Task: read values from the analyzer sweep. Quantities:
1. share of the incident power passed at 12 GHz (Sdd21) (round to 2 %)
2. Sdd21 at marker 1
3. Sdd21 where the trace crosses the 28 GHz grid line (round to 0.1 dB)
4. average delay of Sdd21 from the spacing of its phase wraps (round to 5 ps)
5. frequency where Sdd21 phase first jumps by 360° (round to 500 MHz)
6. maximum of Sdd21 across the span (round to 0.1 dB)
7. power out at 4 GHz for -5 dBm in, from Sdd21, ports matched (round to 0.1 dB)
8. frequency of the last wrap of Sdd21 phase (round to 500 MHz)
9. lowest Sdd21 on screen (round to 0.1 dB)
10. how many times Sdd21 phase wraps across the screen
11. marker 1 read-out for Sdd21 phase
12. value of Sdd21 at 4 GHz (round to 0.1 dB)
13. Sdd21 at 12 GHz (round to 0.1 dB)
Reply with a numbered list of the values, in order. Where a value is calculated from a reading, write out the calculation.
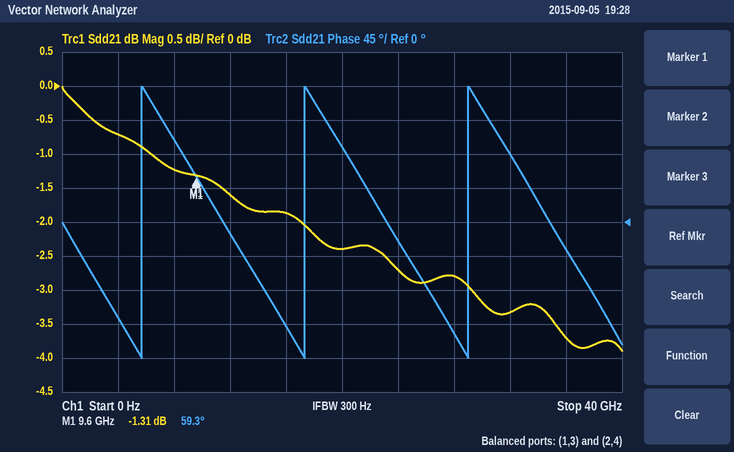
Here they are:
1. 10^(-1.6/10) ≈ 69.2 %, so 70 % to the nearest 2 %
2. -1.31 dB
3. -2.8 dB
4. 2 cycles / (29.0 GHz − 5.5 GHz) ≈ 85 ps
5. 5.5 GHz
6. 0.0 dB
7. -5 dBm + (-0.7 dB) = -5.7 dBm
8. 29.0 GHz
9. -3.9 dB
10. 3
11. 59.3°
12. -0.7 dB
13. -1.6 dB
